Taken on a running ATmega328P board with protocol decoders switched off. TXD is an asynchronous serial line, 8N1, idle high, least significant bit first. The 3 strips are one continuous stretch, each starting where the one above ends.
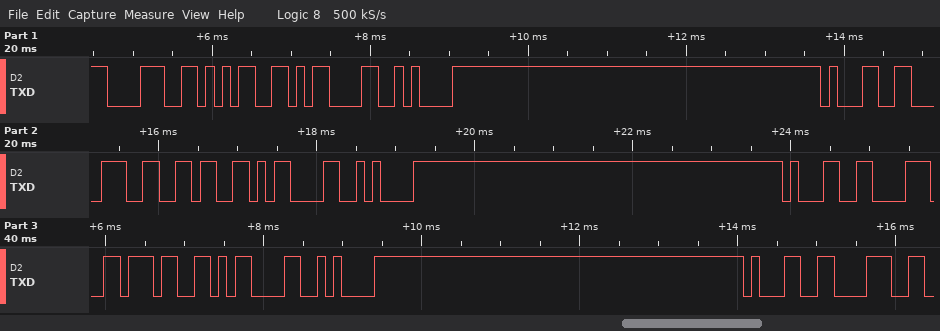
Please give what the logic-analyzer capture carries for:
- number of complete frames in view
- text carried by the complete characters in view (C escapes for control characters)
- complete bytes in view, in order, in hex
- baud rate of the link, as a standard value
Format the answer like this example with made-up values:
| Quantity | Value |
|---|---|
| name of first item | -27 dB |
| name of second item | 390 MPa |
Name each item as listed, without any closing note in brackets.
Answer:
| Quantity | Value |
|---|---|
| number of complete frames in view | 16 |
| text carried by the complete characters in view | "85\r\n186\r\n187\r\n18" |
| complete bytes in view, in order, in hex | 38 35 0D 0A 31 38 36 0D 0A 31 38 37 0D 0A 31 38 |
| baud rate of the link, as a standard value | 9600 baud |
